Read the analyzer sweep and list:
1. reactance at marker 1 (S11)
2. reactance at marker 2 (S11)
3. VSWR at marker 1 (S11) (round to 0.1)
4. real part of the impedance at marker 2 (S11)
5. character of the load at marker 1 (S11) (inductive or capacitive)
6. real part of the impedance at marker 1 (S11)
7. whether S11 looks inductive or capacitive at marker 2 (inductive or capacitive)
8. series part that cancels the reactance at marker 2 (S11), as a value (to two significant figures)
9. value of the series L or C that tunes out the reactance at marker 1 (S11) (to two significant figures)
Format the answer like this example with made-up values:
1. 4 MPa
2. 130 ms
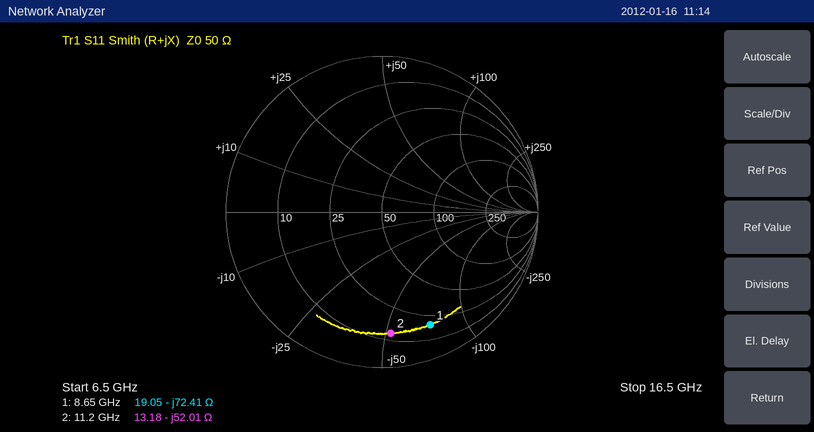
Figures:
1. -72.41 Ω
2. -52.01 Ω
3. 8.4
4. 13.18 Ω
5. capacitive
6. 19.05 Ω
7. capacitive
8. 740 pH
9. 1.3 nH
